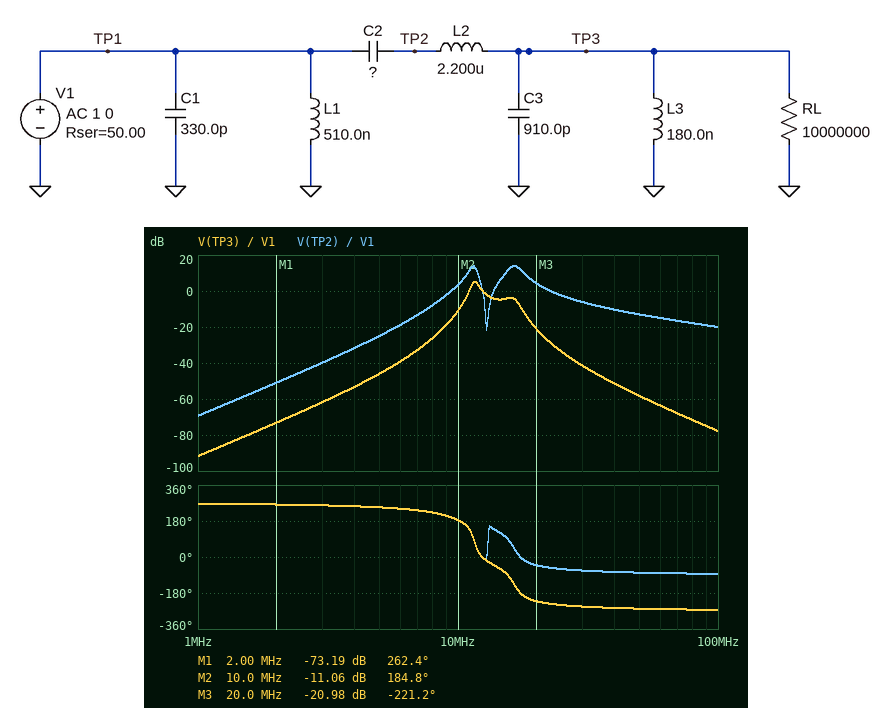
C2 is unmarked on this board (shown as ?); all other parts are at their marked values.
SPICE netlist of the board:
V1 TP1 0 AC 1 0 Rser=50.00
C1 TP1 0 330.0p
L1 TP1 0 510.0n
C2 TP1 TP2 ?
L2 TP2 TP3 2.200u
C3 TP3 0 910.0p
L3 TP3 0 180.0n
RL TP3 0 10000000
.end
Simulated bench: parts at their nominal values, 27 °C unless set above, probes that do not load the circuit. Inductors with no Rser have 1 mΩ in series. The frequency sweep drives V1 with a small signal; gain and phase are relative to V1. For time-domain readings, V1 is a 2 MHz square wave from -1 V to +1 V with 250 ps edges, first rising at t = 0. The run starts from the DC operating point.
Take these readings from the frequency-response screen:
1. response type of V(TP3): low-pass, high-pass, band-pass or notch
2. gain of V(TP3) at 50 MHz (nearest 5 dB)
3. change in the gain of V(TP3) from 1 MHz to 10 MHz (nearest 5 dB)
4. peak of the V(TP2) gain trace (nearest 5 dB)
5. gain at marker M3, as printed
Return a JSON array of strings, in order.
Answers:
["band-pass", "-60 dB", "80 dB", "15 dB", "-20.98 dB"]
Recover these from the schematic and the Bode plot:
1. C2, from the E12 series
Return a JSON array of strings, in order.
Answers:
["56 pF"]
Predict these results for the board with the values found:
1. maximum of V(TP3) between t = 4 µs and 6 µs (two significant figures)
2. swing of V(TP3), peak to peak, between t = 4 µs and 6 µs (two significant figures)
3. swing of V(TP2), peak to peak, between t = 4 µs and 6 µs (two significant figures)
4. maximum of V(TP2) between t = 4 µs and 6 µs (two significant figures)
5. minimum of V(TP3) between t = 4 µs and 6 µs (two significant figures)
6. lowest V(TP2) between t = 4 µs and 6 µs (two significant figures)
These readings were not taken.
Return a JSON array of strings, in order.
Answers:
["190 mV", "390 mV", "2.1 V", "1.0 V", "-190 mV", "-1.0 V"]
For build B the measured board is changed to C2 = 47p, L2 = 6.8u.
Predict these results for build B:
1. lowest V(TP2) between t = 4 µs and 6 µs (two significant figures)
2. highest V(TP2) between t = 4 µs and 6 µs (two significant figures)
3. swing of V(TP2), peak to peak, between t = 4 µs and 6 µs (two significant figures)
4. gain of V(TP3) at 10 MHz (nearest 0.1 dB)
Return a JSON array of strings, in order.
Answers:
["-1.1 V", "1.1 V", "2.2 V", "-14.3 dB"]
